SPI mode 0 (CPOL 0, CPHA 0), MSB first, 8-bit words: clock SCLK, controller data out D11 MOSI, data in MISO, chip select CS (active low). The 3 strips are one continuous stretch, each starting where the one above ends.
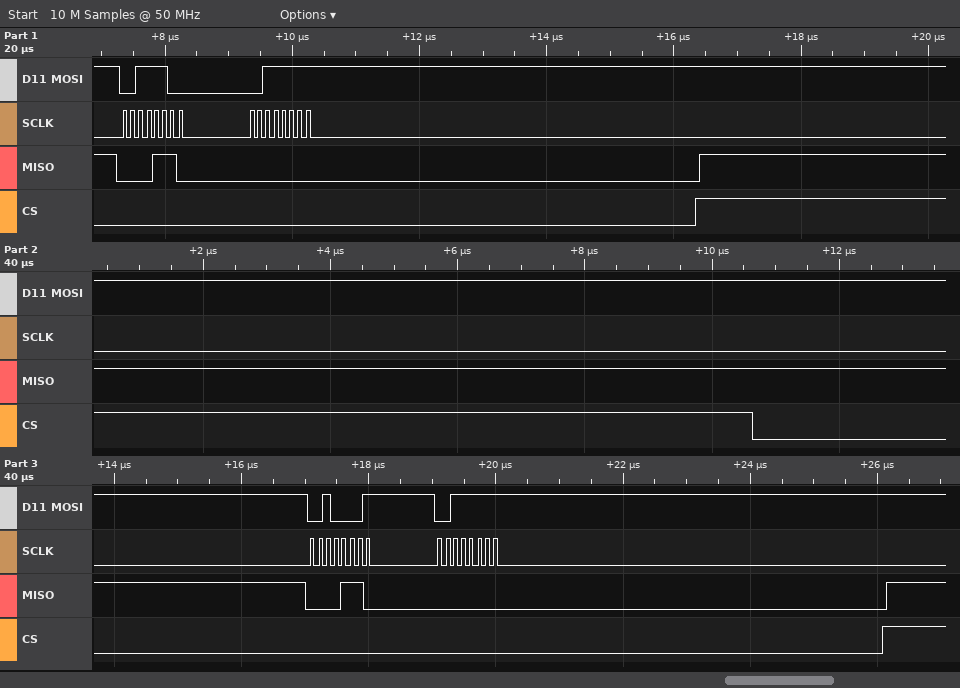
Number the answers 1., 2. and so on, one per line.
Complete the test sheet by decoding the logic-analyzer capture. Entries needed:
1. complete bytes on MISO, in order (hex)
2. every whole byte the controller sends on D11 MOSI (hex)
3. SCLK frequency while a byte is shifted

1. 0E 00 0E 00
2. 3C 3F 21 3F
3. 8 MHz
